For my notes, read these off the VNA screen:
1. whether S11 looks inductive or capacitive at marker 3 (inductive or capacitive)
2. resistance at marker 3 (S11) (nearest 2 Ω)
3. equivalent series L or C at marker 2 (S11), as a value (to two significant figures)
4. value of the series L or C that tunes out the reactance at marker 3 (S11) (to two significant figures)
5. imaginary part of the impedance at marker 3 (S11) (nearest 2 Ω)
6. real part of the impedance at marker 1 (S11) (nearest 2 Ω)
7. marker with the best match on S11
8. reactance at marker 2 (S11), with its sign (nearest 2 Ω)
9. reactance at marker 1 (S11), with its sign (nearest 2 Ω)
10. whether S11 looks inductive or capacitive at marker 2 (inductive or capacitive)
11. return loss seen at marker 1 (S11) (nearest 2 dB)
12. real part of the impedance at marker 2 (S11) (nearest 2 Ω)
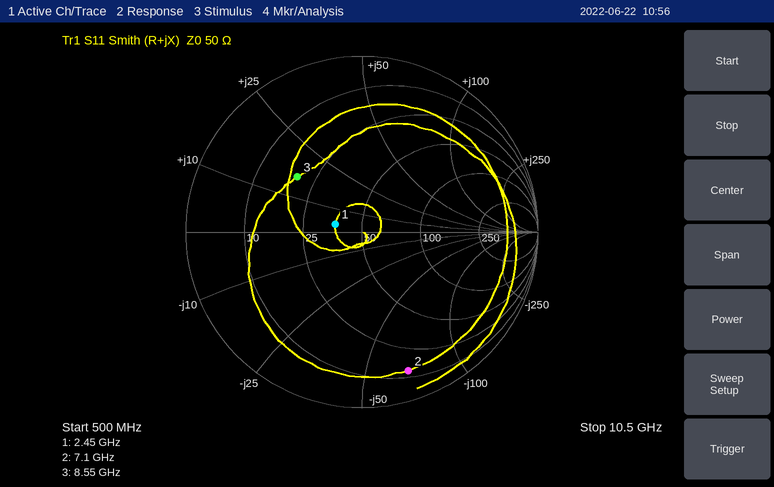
inductive
20 Ω
330 fF
1.2 pF
+16 Ω
36 Ω
marker 1
-68 Ω
+4 Ω
capacitive
16 dB
14 Ω
